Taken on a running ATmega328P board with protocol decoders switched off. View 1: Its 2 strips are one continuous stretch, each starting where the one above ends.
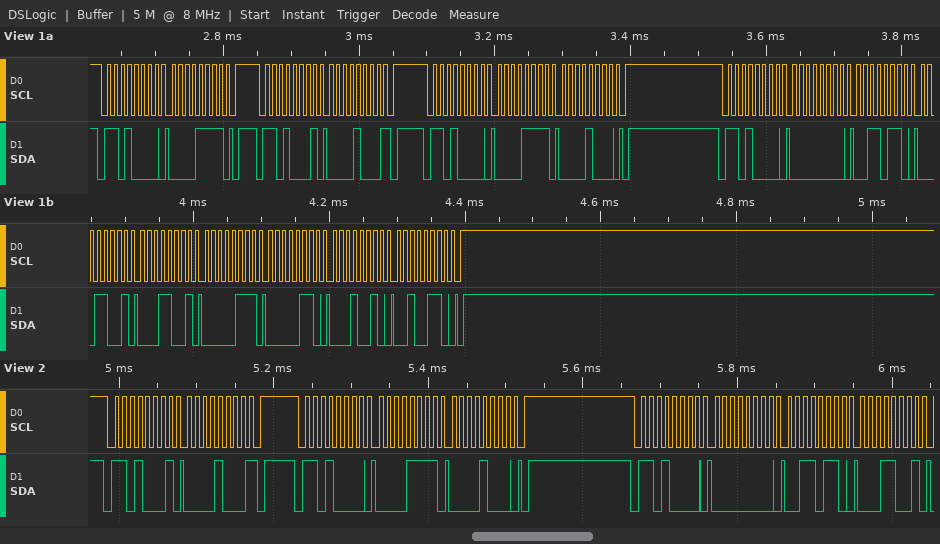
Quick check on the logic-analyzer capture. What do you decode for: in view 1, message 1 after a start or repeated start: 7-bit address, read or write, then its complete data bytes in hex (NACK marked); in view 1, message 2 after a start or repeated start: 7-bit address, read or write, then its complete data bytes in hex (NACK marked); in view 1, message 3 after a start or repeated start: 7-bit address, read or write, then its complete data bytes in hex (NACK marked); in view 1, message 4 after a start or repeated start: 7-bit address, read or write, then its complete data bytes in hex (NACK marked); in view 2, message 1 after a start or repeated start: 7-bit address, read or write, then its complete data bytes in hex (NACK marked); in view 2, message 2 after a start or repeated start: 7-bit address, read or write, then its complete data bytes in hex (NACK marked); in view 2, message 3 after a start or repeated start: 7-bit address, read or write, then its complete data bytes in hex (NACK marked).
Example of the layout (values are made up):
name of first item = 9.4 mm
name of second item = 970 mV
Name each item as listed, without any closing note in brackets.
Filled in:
in view 1, message 1 after a start or repeated start: 7-bit address, read or write, then its complete data bytes in hex = 0x68 write: 0F
in view 1, message 2 after a start or repeated start: 7-bit address, read or write, then its complete data bytes in hex = 0x68 read: 08 NACK
in view 1, message 3 after a start or repeated start: 7-bit address, read or write, then its complete data bytes in hex = 0x68 write: 0F 08
in view 1, message 4 after a start or repeated start: 7-bit address, read or write, then its complete data bytes in hex = 0x68 write: 00 36 19 19 07 06 12 26
in view 2, message 1 after a start or repeated start: 7-bit address, read or write, then its complete data bytes in hex = 0x68 read: 08 NACK
in view 2, message 2 after a start or repeated start: 7-bit address, read or write, then its complete data bytes in hex = 0x68 write: 0F 08
in view 2, message 3 after a start or repeated start: 7-bit address, read or write, then its complete data bytes in hex = 0x68 write: 00 36 19
